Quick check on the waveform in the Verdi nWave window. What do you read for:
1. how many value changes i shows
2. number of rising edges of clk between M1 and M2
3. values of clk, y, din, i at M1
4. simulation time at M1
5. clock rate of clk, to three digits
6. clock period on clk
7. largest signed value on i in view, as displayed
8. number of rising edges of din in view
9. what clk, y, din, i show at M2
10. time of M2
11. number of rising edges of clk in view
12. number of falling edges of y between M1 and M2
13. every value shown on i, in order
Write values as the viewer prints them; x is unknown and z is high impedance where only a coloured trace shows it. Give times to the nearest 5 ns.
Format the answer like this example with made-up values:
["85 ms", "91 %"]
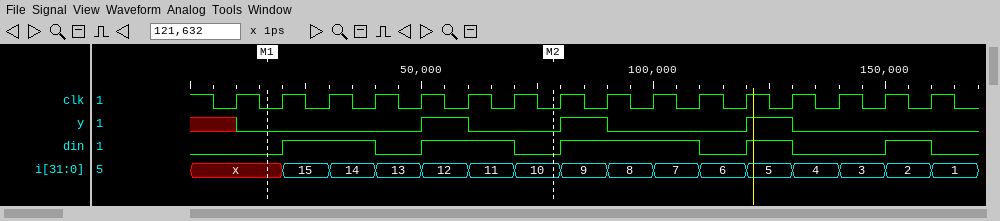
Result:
["15", "6", "clk=0, y=0, din=0, i=x", "15 ns", "100 MHz", "10 ns", "15", "5", "clk=0, y=0, din=0, i=10", "80 ns", "16", "1", "x, 15, 14, 13, 12, 11, 10, 9, 8, 7, 6, 5, 4, 3, 2, 1"]
